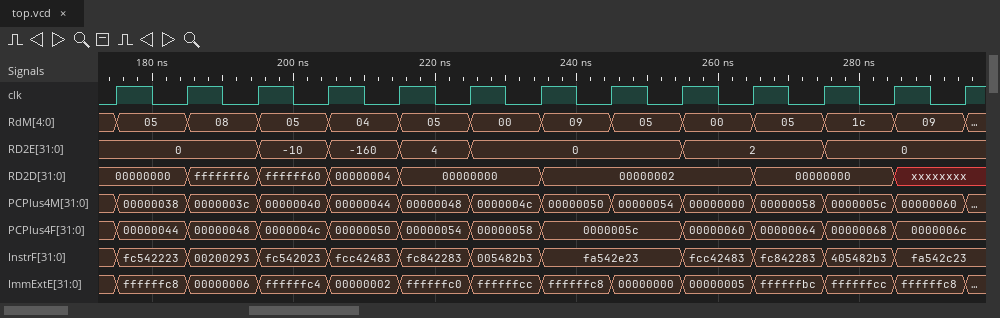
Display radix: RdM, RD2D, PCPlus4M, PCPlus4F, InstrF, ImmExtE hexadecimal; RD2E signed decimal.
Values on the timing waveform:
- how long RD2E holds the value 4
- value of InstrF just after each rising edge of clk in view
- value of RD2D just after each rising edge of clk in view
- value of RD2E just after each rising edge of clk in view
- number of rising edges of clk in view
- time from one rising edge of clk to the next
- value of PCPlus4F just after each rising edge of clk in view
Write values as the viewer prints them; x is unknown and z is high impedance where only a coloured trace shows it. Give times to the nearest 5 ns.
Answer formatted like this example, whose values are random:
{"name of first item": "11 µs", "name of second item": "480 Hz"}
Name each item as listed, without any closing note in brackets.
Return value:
{"how long RD2E holds the value 4": "10 ns", "value of InstrF just after each rising edge of clk in view": "fc542223, 00200293, fc542023, fcc42483, fc842283, 005482b3, fa542e23, fa542e23, fcc42483, fc842283, 405482b3, fa542c23, fa542c23", "value of RD2D just after each rising edge of clk in view": "00000000, fffffff6, ffffff60, 00000004, 00000000, 00000000, 00000002, 00000002, 00000002, 00000000, 00000000, xxxxxxxx, xxxxxxxx", "value of RD2E just after each rising edge of clk in view": "0, 0, -10, -160, 4, 0, 0, 0, 2, 2, 0, 0, 0", "number of rising edges of clk in view": "13", "time from one rising edge of clk to the next": "10 ns", "value of PCPlus4F just after each rising edge of clk in view": "00000044, 00000048, 0000004c, 00000050, 00000054, 00000058, 0000005c, 0000005c, 00000060, 00000064, 00000068, 0000006c, 0000006c"}
